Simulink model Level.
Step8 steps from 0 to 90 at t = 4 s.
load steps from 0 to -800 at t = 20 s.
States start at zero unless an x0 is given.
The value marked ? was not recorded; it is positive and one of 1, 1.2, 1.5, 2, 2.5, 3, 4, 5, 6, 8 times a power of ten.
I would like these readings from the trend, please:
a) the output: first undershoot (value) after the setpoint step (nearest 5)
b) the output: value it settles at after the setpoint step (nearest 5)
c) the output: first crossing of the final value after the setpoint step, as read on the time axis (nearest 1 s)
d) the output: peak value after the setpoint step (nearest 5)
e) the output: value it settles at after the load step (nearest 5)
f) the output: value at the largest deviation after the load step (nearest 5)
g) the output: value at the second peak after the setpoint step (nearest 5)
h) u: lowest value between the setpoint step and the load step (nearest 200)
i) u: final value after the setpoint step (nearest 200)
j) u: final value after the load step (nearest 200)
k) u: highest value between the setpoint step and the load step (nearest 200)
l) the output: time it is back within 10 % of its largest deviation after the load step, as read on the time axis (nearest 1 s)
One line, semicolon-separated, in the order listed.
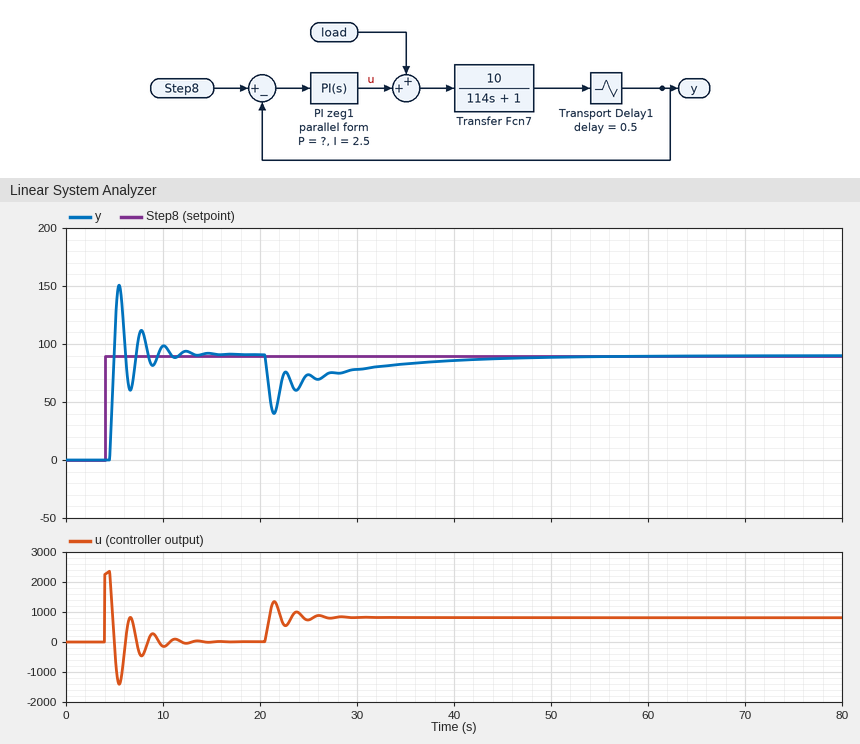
60; 90; 5 s; 150; 90; 40; 110; -1400; 0; 800; 2400; 38 s
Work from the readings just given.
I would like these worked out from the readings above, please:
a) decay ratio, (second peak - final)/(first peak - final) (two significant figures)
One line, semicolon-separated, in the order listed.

0.33
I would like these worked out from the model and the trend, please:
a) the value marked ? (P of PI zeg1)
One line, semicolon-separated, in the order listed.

25
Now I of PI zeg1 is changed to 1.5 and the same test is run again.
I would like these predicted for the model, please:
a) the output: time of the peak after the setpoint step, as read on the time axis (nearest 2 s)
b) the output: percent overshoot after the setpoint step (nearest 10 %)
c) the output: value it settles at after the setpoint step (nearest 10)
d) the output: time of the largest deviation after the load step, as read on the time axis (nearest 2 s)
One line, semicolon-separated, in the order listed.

6 s; 60 %; 90; 22 s
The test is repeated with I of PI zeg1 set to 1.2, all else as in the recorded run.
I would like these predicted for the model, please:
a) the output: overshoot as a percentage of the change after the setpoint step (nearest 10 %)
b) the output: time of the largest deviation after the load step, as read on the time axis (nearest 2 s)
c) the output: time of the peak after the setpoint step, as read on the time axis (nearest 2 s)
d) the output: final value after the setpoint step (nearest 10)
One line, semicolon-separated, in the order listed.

60 %; 22 s; 6 s; 90
